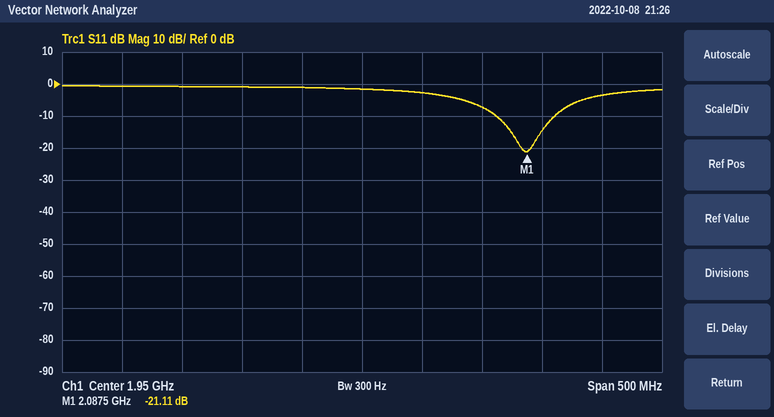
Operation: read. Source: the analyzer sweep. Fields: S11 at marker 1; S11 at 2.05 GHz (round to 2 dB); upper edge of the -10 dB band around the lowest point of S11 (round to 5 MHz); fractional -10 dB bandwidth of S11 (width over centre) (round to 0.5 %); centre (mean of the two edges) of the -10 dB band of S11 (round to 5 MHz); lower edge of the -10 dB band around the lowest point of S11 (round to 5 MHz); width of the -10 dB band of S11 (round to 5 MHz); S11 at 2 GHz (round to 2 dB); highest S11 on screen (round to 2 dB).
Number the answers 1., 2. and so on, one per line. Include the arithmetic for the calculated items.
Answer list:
1. -21.11 dB
2. -8 dB
3. 2.110 GHz
4. 50 MHz / 2.085 GHz ≈ 2.40 %, so 2.5 % to the nearest 0.5 %
5. 2.085 GHz
6. 2.060 GHz
7. 2.110 GHz − 2.060 GHz = 50 MHz
8. -2 dB
9. 0 dB
